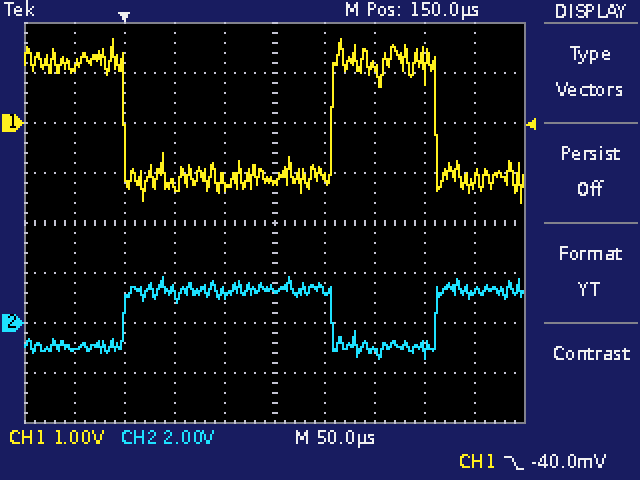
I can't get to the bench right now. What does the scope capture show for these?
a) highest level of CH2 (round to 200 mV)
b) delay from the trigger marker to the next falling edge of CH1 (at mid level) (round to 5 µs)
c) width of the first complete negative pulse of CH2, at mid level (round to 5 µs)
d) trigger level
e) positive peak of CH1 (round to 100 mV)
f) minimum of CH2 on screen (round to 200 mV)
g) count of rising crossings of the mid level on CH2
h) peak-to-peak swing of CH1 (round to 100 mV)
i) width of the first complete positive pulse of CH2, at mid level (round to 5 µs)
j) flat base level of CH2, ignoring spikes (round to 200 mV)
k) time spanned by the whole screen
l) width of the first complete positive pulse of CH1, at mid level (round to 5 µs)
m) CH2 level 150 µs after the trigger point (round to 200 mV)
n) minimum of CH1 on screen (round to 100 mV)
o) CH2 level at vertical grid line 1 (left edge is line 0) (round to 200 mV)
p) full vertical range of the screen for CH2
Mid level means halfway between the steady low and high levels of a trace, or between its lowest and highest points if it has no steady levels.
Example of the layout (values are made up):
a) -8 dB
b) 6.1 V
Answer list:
a) 1.8 V
b) 310 µs
c) 105 µs
d) -40.0 mV
e) 1.7 V
f) -1.4 V
g) 2
h) 3.3 V
i) 210 µs
j) -1.0 V
k) 500 µs
l) 105 µs
m) 1.4 V
n) -1.6 V
o) -1.0 V
p) 16 V
